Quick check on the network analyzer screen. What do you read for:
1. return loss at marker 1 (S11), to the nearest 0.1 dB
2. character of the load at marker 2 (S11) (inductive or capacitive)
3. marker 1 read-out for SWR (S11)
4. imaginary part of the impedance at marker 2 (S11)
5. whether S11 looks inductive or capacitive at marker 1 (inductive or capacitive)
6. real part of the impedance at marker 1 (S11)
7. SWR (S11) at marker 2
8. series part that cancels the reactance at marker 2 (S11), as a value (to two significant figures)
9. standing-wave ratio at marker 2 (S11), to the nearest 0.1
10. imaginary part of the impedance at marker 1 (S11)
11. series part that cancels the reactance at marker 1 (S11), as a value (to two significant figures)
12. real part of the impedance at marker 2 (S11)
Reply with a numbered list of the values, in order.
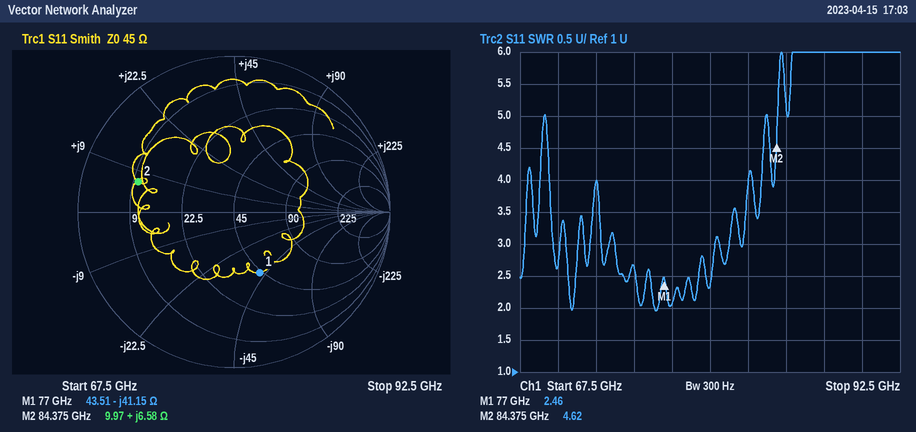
1. 7.5 dB
2. inductive
3. 2.46
4. +6.58 Ω
5. capacitive
6. 43.51 Ω
7. 4.62
8. 290 fF
9. 4.6
10. -41.15 Ω
11. 85 pH
12. 9.97 Ω
